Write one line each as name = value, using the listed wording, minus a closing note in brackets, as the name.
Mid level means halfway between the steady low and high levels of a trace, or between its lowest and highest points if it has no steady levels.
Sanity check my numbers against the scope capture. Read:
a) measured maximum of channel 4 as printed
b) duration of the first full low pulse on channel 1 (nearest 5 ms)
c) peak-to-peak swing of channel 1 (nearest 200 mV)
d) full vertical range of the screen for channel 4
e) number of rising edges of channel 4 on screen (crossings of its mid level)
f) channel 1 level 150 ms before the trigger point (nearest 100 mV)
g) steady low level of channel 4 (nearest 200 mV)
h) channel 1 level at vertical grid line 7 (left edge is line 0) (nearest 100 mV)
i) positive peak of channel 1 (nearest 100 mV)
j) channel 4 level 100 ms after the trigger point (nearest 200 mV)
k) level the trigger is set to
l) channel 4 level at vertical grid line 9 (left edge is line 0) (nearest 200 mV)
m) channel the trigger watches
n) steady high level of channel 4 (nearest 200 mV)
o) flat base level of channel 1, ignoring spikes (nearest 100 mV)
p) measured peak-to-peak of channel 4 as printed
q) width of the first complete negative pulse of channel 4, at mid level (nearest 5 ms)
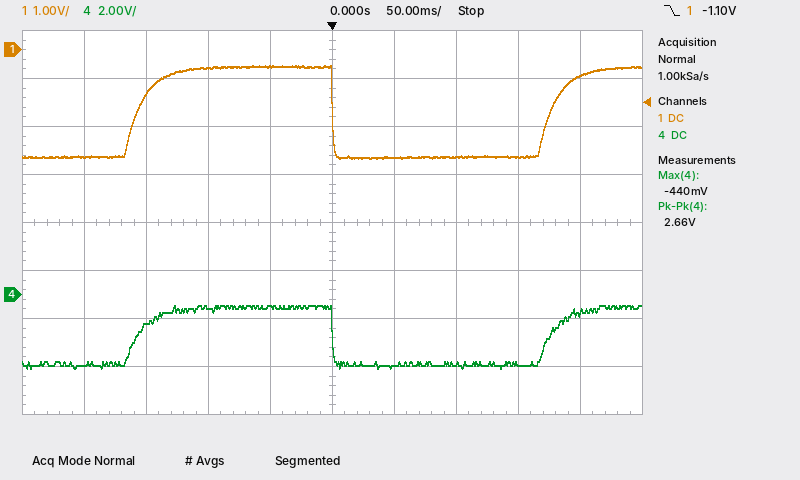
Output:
measured maximum of channel 4 as printed = -440 mV
duration of the first full low pulse on channel 1 = 175 ms
peak-to-peak swing of channel 1 = 2.0 V
full vertical range of the screen for channel 4 = 16 V
number of rising edges of channel 4 on screen = 2
channel 1 level 150 ms before the trigger point = -900 mV
steady low level of channel 4 = -3.0 V
channel 1 level at vertical grid line 7 (left edge is line 0) = -2.2 V
positive peak of channel 1 = -300 mV
channel 4 level 100 ms after the trigger point = -2.8 V
level the trigger is set to = -1.10 V
channel 4 level at vertical grid line 9 (left edge is line 0) = -800 mV
channel the trigger watches = channel 1
steady high level of channel 4 = -600 mV
flat base level of channel 1, ignoring spikes = -2.2 V
measured peak-to-peak of channel 4 as printed = 2.66 V
width of the first complete negative pulse of channel 4, at mid level = 175 ms
